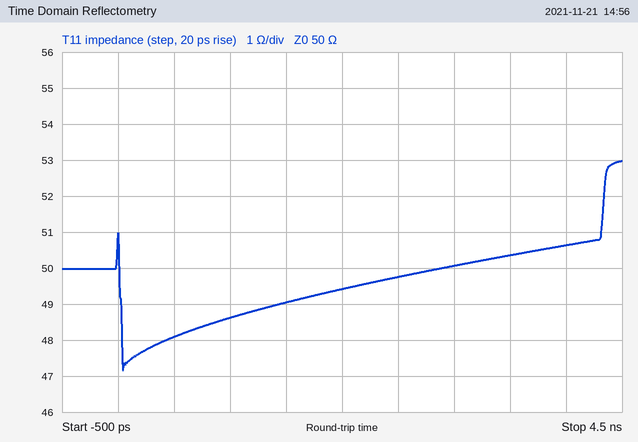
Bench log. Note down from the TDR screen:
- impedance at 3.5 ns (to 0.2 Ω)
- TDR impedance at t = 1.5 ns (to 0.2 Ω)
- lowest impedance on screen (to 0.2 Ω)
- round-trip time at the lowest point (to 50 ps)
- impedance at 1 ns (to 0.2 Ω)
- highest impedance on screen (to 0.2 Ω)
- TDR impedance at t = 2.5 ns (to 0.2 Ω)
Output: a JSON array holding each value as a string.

["50.4 Ω", "49.0 Ω", "47.2 Ω", "50 ps", "48.6 Ω", "53.0 Ω", "49.8 Ω"]
